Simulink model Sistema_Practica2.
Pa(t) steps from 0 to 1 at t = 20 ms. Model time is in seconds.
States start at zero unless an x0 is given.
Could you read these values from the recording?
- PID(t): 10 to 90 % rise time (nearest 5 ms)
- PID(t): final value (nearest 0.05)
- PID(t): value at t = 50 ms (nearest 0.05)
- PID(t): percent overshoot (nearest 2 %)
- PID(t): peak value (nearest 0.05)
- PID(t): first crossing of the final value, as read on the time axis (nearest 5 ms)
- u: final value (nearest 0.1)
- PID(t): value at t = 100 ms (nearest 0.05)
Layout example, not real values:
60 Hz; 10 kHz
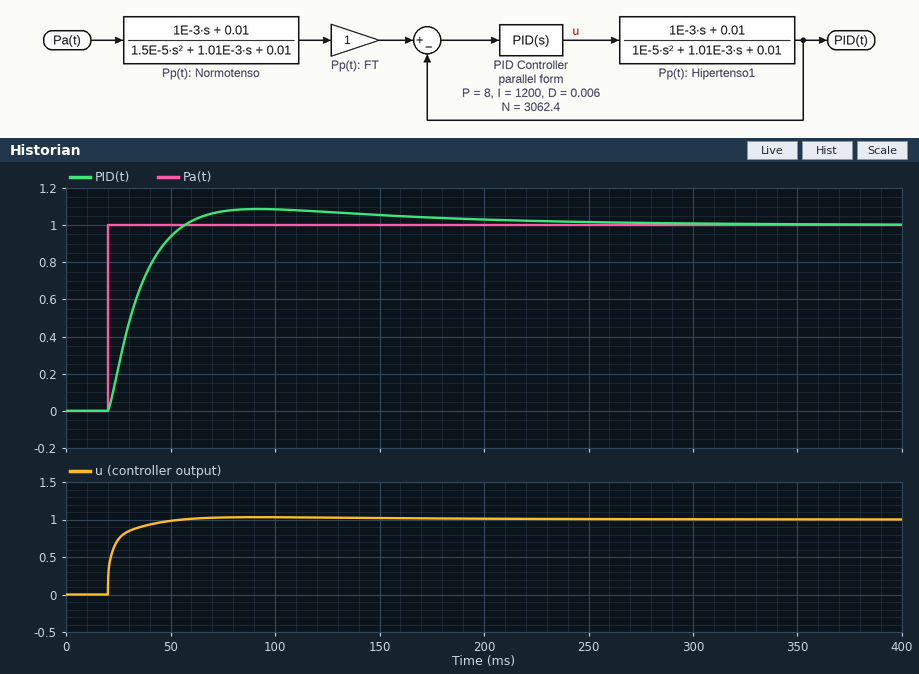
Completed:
25 ms; 1.00; 0.95; 8 %; 1.10; 55 ms; 1.0; 1.10
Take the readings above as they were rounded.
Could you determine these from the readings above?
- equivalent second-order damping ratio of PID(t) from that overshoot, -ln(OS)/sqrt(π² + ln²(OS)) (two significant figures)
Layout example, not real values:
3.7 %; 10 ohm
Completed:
0.63
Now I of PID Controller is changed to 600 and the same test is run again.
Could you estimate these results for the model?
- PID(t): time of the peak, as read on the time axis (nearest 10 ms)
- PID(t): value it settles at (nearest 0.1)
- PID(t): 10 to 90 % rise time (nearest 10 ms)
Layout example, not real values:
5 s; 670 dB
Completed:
90 ms; 1.0; 30 ms
